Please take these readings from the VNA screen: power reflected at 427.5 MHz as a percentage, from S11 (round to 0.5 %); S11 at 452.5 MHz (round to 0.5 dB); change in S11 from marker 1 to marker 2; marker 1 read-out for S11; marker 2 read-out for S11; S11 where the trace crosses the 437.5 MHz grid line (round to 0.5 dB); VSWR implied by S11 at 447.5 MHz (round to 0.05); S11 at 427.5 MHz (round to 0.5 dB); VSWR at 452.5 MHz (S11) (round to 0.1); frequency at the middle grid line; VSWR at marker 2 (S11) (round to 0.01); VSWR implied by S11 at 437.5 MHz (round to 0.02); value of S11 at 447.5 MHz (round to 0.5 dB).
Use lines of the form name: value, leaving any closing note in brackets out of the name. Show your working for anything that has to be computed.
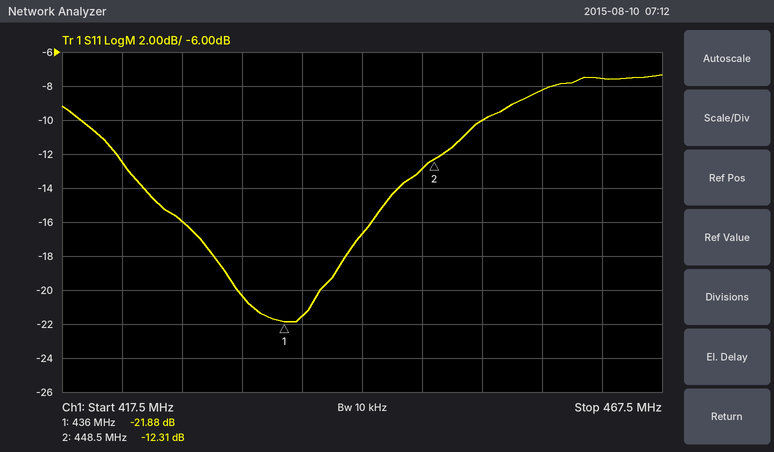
power reflected at 427.5 MHz as a percentage, from S11: 10^(-16/10) ≈ 2.5 %
S11 at 452.5 MHz: -10.0 dB
change in S11 from marker 1 to marker 2: -12.31 − (-21.88) = 9.57 dB
marker 1 read-out for S11: -21.88 dB
marker 2 read-out for S11: -12.31 dB
S11 where the trace crosses the 437.5 MHz grid line: -21.5 dB
VSWR implied by S11 at 447.5 MHz: |Γ| = 10^(-13/20) = 0.2239; VSWR = (1 + 0.2239)/(1 − 0.2239) ≈ 1.58, so 1.60 to the nearest 0.05
S11 at 427.5 MHz: -16.0 dB
VSWR at 452.5 MHz (S11): |Γ| = 10^(-10/20) = 0.3162; VSWR = (1 + 0.3162)/(1 − 0.3162) ≈ 1.9
frequency at the middle grid line: 442.5 MHz
VSWR at marker 2 (S11): (1 + 0.2424)/(1 − 0.2424) ≈ 1.64
VSWR implied by S11 at 437.5 MHz: |Γ| = 10^(-21.5/20) = 0.0841; VSWR = (1 + 0.0841)/(1 − 0.0841) ≈ 1.18
value of S11 at 447.5 MHz: -13.0 dB
